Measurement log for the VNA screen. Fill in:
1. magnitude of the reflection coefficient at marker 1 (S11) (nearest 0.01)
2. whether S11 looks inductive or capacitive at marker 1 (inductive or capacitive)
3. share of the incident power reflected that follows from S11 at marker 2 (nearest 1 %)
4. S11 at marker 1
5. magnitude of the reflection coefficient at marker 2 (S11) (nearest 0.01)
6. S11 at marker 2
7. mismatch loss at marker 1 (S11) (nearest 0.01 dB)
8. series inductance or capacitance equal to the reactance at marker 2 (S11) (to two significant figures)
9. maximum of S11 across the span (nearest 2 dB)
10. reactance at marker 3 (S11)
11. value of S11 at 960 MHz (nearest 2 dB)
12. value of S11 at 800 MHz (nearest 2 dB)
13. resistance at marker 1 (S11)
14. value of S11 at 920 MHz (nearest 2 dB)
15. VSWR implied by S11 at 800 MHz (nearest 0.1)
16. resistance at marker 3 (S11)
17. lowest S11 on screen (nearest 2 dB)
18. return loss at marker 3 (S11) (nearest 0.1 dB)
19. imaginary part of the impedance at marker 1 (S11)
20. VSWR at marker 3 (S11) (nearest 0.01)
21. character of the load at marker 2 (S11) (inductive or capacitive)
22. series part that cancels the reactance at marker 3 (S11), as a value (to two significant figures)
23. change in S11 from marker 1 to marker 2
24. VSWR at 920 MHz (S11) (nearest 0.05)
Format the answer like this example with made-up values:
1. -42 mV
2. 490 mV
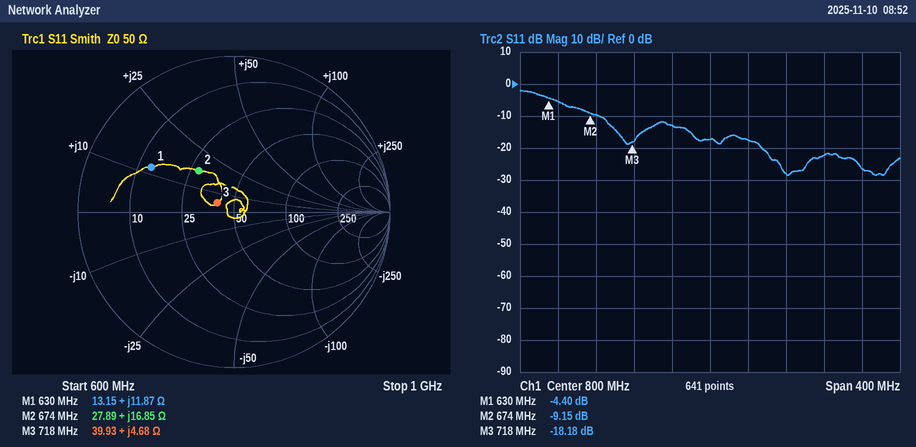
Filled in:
1. 0.60
2. inductive
3. 12 %
4. -4.40 dB
5. 0.35
6. -9.15 dB
7. 1.96 dB
8. 4.0 nH
9. -2 dB
10. +4.68 Ω
11. -26 dB
12. -18 dB
13. 13.15 Ω
14. -22 dB
15. 1.3
16. 39.93 Ω
17. -28 dB
18. 18.2 dB
19. +11.87 Ω
20. 1.28
21. inductive
22. 47 pF
23. -4.75 dB
24. 1.15
